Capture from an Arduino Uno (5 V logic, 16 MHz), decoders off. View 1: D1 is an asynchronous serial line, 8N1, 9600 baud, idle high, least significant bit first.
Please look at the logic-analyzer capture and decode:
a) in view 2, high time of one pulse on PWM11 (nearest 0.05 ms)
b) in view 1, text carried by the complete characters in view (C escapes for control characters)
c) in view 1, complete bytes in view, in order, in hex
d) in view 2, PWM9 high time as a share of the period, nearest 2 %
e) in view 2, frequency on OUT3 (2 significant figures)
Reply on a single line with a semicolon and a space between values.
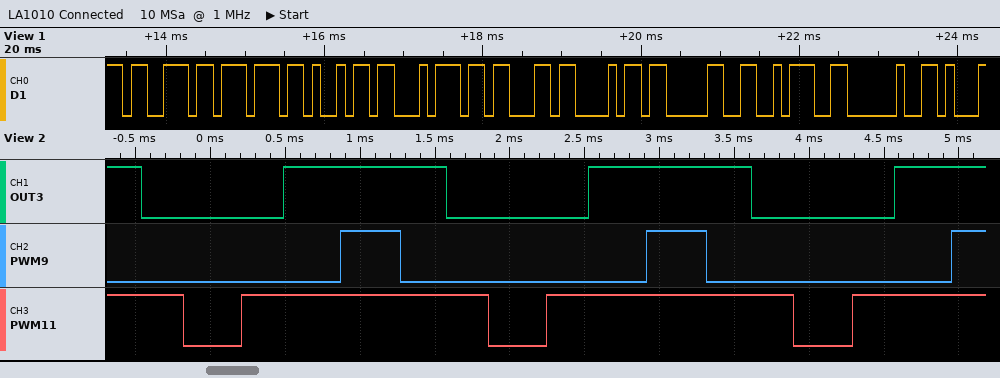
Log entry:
1.65 ms; "switch0: "; 73 77 69 74 63 68 30 3A 20; 20 %; 490 Hz
